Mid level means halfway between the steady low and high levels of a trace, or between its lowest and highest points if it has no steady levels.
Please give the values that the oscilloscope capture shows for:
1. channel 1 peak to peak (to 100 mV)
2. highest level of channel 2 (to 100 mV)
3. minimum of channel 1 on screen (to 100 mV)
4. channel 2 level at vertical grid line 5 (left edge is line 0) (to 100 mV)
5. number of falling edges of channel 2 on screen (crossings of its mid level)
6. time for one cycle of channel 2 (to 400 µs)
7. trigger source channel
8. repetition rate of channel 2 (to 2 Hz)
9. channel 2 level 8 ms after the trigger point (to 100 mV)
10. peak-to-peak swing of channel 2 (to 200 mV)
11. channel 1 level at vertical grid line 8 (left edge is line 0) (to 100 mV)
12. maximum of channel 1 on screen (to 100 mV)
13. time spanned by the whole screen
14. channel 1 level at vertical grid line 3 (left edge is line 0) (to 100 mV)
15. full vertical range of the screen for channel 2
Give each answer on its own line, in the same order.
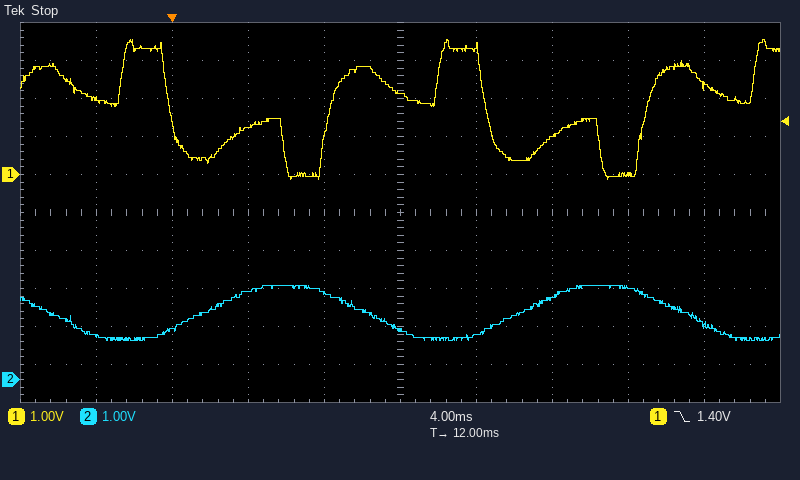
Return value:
3.7 V
2.5 V
-100 mV
1.3 V
3
16.8 ms
channel 1
60 Hz
2.3 V
1.4 V
0.0 V
3.6 V
40 ms
1.3 V
10 V
